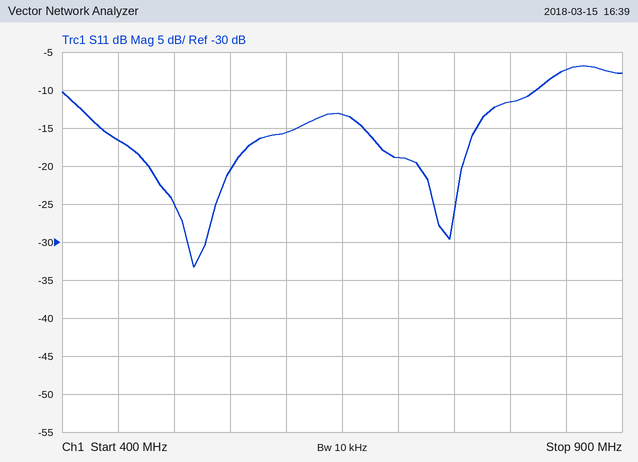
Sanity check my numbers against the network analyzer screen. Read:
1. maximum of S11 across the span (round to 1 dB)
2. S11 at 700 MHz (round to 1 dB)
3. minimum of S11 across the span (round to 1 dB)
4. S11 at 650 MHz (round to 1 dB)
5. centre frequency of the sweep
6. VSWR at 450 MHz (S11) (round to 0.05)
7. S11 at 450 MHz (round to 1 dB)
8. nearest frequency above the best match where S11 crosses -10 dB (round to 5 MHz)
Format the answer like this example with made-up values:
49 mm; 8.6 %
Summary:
-7 dB; -19 dB; -33 dB; -13 dB; 650 MHz; 1.35; -17 dB; 825 MHz
